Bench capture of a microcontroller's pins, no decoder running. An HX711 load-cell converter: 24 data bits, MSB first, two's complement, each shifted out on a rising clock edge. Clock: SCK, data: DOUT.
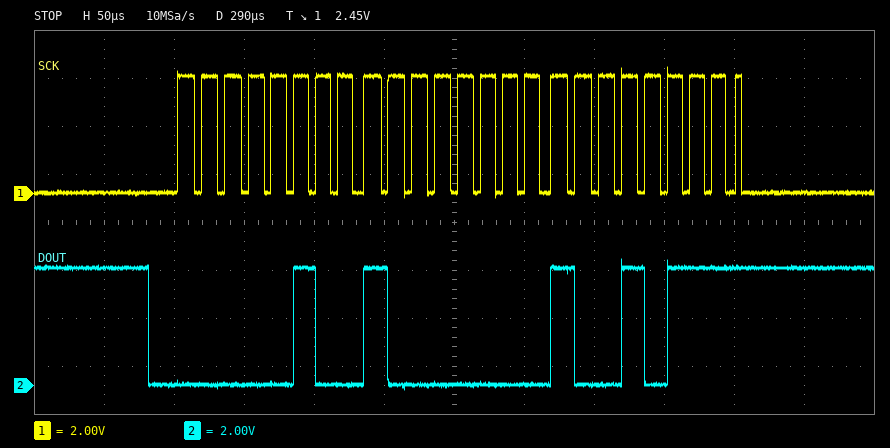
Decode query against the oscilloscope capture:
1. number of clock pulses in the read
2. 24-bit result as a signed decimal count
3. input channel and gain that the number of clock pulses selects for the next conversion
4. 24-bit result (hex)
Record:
25
295063
channel A, gain 128
0x048097
